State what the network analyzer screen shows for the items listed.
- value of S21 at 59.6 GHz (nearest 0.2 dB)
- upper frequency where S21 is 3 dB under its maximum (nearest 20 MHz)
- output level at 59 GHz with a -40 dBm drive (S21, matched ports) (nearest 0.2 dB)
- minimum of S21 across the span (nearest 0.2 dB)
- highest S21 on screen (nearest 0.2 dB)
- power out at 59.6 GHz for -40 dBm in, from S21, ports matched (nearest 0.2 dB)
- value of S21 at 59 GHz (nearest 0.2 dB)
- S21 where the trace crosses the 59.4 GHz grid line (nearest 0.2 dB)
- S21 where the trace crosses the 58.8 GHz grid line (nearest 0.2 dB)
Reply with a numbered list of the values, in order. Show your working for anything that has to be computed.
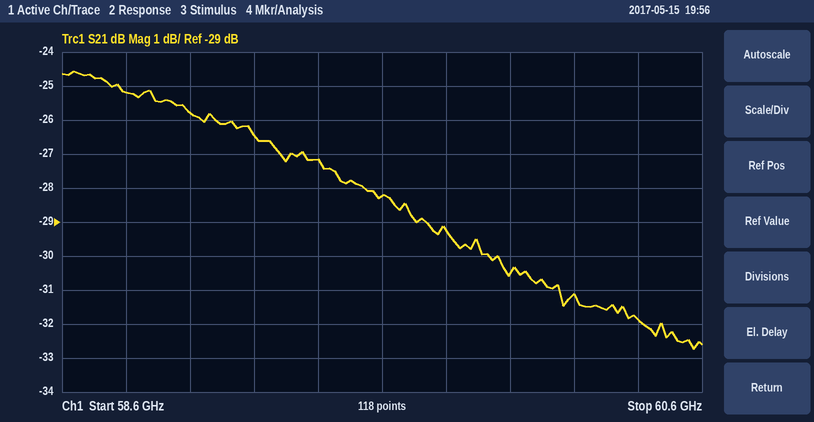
1. -28.2 dB
2. 59.46 GHz
3. -40 dBm + (-25.8 dB) = -65.8 dBm
4. -32.8 dB
5. -24.6 dB
6. -40 dBm + (-28.2 dB) = -68.2 dBm
7. -25.8 dB
8. -27.2 dB
9. -25.2 dB
